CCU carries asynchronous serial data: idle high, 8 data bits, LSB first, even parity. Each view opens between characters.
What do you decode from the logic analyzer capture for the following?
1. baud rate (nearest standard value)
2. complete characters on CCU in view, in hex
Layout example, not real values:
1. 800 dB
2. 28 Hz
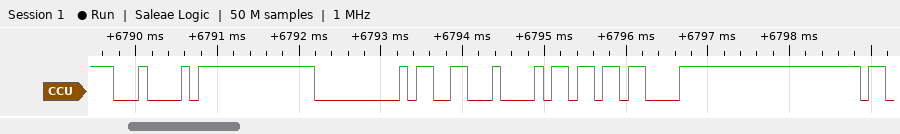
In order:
1. 9600 baud
2. 84, 00, 33, 68, 1B
